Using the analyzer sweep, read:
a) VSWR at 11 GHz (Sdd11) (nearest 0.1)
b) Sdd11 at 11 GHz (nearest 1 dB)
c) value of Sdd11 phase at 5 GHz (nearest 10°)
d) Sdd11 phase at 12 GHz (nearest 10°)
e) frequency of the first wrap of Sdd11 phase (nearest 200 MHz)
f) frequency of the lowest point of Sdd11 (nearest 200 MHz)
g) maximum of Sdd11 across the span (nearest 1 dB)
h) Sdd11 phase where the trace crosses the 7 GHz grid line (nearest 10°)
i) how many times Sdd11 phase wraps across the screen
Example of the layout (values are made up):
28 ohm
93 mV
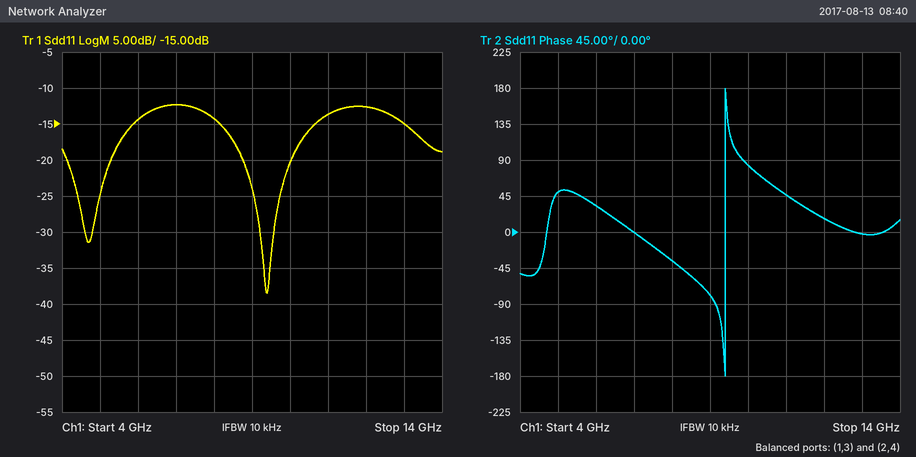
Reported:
1.5
-14 dB
50°
20°
9.4 GHz
9.4 GHz
-12 dB
0°
1
